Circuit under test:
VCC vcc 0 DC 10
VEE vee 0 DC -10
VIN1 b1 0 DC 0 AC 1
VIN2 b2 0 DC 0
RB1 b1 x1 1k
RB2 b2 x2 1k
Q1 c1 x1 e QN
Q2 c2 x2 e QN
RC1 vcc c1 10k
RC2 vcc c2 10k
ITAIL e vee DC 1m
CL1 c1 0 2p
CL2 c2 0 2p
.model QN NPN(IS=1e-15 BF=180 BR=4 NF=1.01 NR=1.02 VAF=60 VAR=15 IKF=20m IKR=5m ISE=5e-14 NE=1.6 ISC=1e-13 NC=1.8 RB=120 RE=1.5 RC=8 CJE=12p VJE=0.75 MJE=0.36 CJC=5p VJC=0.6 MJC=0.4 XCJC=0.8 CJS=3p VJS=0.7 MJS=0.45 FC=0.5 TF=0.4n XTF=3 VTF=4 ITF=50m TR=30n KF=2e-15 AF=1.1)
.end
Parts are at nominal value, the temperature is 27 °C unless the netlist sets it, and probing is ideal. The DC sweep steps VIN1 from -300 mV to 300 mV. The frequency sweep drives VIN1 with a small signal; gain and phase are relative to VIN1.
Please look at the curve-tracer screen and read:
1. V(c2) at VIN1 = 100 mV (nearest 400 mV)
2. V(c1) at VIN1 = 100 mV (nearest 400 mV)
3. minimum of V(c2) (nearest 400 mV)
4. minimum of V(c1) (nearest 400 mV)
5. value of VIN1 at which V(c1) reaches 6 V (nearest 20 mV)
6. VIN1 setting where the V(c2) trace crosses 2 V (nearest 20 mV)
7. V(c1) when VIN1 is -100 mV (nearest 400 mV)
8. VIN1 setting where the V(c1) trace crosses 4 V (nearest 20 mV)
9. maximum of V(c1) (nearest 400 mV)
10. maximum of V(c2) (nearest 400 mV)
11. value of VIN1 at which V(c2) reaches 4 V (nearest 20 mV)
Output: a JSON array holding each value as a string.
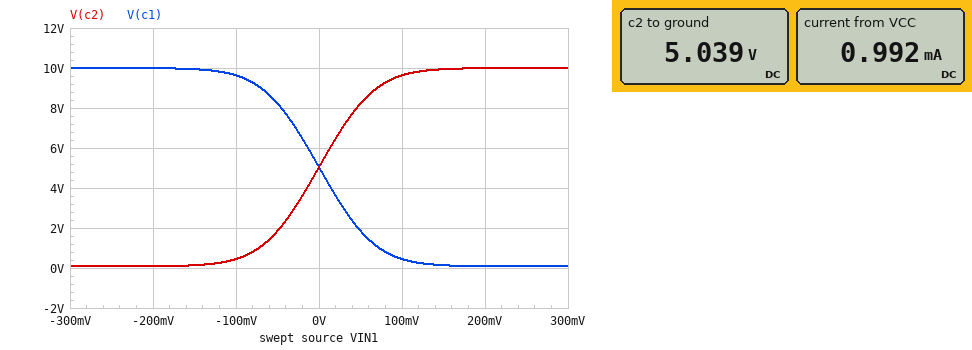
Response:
["9.6 V", "400 mV", "0 V", "0 V", "-20 mV", "-40 mV", "9.6 V", "20 mV", "10.0 V", "10.0 V", "-20 mV"]
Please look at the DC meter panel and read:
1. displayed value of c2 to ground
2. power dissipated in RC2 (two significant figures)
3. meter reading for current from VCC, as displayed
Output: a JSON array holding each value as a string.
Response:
["5.039 V", "2.5 mW", "0.992 mA"]
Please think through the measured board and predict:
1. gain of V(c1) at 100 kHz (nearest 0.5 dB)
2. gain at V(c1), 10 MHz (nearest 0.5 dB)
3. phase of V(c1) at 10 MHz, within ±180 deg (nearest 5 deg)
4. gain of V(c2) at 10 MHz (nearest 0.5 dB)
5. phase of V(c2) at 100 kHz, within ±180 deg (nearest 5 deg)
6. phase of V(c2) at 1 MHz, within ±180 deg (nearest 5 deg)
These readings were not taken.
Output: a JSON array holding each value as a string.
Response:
["37.0 dB", "9.5 dB", "75 deg", "9.0 dB", "-15 deg", "-70 deg"]
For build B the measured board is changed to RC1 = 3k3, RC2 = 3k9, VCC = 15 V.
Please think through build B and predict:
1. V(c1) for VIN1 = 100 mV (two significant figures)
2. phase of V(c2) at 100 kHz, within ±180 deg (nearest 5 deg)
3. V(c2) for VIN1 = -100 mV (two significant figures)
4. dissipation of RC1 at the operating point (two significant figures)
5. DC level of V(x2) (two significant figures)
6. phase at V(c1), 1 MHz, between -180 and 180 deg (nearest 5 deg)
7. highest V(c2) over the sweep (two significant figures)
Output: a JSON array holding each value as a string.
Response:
["12 V", "-5 deg", "11 V", "820 µW", "-3.5 mV", "140 deg", "15 V"]
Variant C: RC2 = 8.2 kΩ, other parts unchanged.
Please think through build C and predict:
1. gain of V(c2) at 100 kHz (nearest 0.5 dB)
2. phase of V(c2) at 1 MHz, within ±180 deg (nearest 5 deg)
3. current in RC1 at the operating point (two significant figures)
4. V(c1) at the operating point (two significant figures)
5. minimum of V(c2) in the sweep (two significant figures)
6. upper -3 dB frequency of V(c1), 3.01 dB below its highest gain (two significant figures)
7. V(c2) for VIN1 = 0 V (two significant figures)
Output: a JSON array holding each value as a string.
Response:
["35.5 dB", "-65 deg", "490 µA", "5.1 V", "1.9 V", "440 kHz", "5.9 V"]
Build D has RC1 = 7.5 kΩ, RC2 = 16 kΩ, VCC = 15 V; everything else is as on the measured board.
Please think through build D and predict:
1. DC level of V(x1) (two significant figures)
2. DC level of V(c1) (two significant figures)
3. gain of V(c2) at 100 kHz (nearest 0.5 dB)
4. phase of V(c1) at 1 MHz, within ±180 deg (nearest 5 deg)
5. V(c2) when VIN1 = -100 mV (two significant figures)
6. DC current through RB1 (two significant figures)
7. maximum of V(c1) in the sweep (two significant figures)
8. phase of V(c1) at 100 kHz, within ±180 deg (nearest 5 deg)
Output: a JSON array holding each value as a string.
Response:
["-3.7 mV", "11 V", "41.0 dB", "120 deg", "-230 mV", "3.7 µA", "15 V", "165 deg"]
